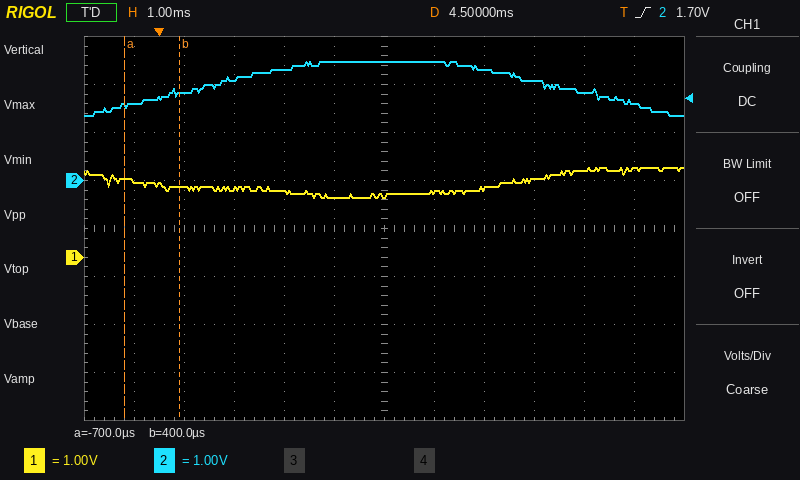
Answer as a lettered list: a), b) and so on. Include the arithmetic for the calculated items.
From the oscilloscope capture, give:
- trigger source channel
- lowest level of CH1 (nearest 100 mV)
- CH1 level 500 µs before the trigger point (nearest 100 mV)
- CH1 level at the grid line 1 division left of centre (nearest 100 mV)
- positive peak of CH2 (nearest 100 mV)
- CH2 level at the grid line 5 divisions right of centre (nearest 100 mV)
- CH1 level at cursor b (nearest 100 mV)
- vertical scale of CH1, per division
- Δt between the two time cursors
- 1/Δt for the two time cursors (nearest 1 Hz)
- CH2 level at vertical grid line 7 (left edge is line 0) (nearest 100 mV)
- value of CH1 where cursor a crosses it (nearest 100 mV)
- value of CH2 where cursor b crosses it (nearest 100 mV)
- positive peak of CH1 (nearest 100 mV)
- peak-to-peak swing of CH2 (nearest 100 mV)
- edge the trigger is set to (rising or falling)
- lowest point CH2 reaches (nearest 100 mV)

a) CH2
b) 1.2 V
c) 1.6 V
d) 1.2 V
e) 2.5 V
f) 1.6 V
g) 1.5 V
h) 1 V
i) 400 µs − (-700 µs) = 1.1 ms
j) 1 / 1.1 ms ≈ 909 Hz
k) 2.5 V
l) 1.6 V
m) 1.8 V
n) 1.9 V
o) 2.5 V − (1.4 V) = 1.1 V
p) rising
q) 1.4 V
